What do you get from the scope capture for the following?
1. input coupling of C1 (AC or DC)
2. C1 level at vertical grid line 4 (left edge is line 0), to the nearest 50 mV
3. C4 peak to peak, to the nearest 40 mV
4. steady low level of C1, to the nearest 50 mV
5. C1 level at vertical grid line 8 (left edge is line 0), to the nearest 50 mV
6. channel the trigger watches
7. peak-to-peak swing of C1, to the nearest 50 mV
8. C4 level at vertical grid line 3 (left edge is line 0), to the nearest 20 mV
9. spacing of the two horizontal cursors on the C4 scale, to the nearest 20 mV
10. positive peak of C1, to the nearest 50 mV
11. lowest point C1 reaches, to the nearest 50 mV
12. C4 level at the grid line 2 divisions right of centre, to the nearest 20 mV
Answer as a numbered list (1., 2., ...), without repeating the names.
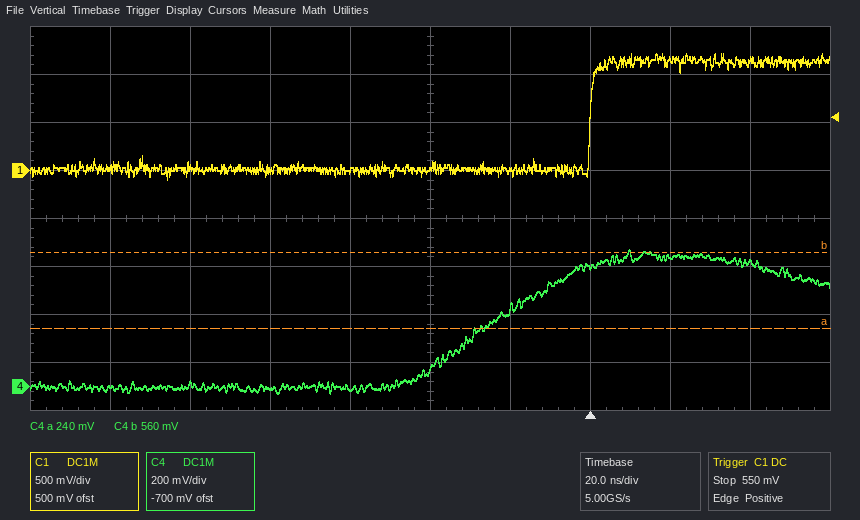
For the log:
1. DC
2. 0 mV
3. 600 mV
4. 0 mV
5. 1.15 V
6. C1
7. 1.30 V
8. 0 mV
9. 320 mV
10. 1.20 V
11. -100 mV
12. 500 mV
